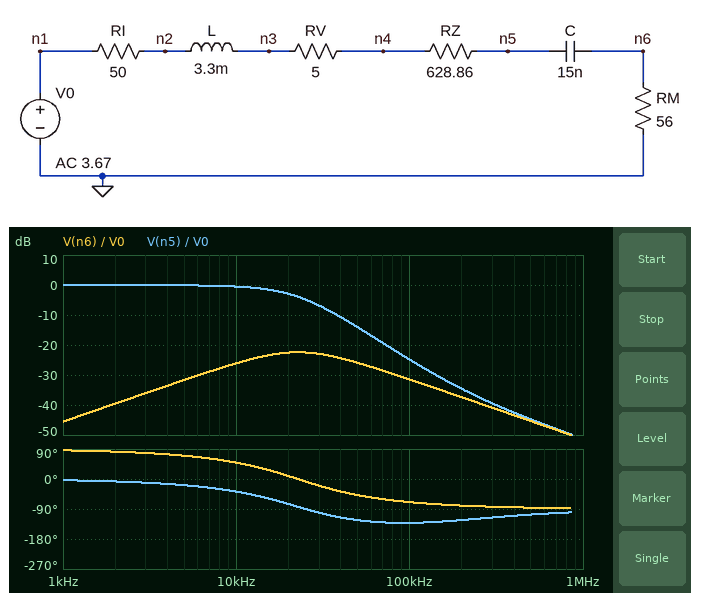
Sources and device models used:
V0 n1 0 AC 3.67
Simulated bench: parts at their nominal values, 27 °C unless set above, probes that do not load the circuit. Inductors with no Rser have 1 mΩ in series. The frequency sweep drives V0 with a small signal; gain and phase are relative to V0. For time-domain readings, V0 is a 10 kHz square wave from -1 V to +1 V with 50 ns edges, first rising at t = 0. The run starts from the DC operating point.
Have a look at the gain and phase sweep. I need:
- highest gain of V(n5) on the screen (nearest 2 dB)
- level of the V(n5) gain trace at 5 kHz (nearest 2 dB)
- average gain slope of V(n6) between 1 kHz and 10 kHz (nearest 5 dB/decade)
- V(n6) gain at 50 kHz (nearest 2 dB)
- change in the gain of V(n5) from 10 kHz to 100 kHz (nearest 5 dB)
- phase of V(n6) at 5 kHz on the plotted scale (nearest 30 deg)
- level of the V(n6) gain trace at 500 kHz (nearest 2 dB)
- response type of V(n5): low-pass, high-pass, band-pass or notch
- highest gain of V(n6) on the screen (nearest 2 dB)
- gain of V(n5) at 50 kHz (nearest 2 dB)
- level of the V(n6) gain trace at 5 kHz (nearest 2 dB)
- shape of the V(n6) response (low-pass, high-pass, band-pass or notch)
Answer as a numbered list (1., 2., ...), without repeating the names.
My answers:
1. 0 dB
2. 0 dB
3. 20 dB/decade
4. -26 dB
5. -25 dB
6. 60 deg
7. -46 dB
8. low-pass
9. -22 dB
10. -14 dB
11. -32 dB
12. band-pass
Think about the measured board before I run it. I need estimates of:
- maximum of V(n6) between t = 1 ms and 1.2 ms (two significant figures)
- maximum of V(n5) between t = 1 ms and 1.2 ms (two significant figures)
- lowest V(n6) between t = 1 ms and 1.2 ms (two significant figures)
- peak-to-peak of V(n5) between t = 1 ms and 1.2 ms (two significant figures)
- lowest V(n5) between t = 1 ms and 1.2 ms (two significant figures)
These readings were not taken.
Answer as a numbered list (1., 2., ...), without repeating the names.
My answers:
1. 100 mV
2. 1.0 V
3. -100 mV
4. 2.1 V
5. -1.0 V
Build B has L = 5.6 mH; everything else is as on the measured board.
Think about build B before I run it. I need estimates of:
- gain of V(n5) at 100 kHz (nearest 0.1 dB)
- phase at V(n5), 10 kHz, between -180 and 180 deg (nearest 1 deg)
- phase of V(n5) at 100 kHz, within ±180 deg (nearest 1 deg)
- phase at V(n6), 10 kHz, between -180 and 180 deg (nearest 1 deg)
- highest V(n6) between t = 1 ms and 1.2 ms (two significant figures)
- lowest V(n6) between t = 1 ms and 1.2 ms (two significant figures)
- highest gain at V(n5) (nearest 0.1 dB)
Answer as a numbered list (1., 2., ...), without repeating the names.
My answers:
1. -29.3 dB
2. -43 deg
3. -140 deg
4. 44 deg
5. 95 mV
6. -95 mV
7. 0.3 dB
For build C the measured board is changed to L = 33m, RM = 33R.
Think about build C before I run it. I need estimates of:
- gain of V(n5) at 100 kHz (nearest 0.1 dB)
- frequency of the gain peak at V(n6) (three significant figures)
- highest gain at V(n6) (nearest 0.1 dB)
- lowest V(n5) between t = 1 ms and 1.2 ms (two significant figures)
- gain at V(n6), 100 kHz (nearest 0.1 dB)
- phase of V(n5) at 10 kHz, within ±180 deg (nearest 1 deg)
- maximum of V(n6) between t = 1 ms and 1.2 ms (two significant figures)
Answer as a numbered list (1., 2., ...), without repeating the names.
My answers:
1. -45.4 dB
2. 7.15 kHz
3. -26.7 dB
4. -1.1 V
5. -55.9 dB
6. -143 deg
7. 33 mV
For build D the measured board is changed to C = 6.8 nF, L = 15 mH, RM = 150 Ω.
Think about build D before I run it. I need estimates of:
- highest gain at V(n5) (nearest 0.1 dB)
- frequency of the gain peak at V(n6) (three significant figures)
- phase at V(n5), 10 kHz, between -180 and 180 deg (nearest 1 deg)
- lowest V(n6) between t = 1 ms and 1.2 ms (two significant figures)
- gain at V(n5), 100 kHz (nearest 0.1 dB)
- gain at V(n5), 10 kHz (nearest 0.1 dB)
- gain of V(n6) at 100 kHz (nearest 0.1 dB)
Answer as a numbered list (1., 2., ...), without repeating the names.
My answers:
1. 5.4 dB
2. 15.8 kHz
3. -27 deg
4. -140 mV
5. -30.4 dB
6. 3.2 dB
7. -35.8 dB
